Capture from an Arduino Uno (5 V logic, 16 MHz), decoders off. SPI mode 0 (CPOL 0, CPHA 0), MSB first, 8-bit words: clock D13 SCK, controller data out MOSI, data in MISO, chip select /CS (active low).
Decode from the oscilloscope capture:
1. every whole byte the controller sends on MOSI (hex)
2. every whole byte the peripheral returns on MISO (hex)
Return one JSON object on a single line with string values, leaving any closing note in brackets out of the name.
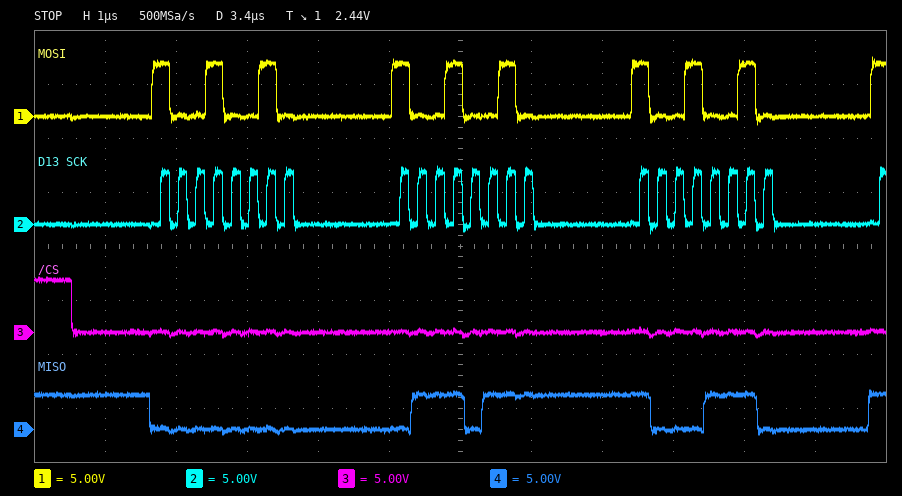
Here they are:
{"every whole byte the controller sends on MOSI": "92 92 92", "every whole byte the peripheral returns on MISO": "00 77 8E"}
